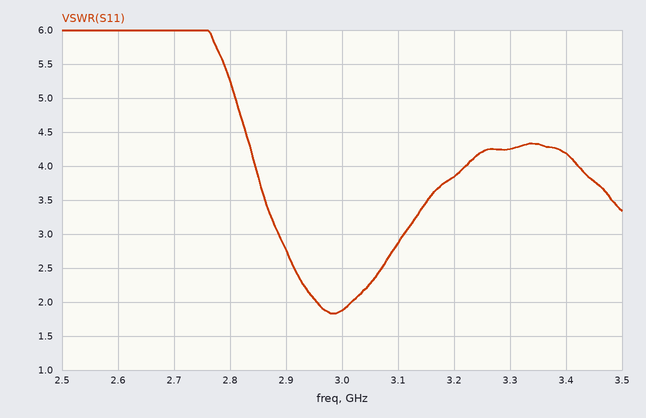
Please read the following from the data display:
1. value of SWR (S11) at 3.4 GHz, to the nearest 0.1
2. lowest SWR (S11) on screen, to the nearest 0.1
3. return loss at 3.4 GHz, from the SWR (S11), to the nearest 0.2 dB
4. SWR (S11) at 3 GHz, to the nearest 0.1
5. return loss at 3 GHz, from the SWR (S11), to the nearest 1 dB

4.2
1.8
4.2 dB
1.9
10 dB
